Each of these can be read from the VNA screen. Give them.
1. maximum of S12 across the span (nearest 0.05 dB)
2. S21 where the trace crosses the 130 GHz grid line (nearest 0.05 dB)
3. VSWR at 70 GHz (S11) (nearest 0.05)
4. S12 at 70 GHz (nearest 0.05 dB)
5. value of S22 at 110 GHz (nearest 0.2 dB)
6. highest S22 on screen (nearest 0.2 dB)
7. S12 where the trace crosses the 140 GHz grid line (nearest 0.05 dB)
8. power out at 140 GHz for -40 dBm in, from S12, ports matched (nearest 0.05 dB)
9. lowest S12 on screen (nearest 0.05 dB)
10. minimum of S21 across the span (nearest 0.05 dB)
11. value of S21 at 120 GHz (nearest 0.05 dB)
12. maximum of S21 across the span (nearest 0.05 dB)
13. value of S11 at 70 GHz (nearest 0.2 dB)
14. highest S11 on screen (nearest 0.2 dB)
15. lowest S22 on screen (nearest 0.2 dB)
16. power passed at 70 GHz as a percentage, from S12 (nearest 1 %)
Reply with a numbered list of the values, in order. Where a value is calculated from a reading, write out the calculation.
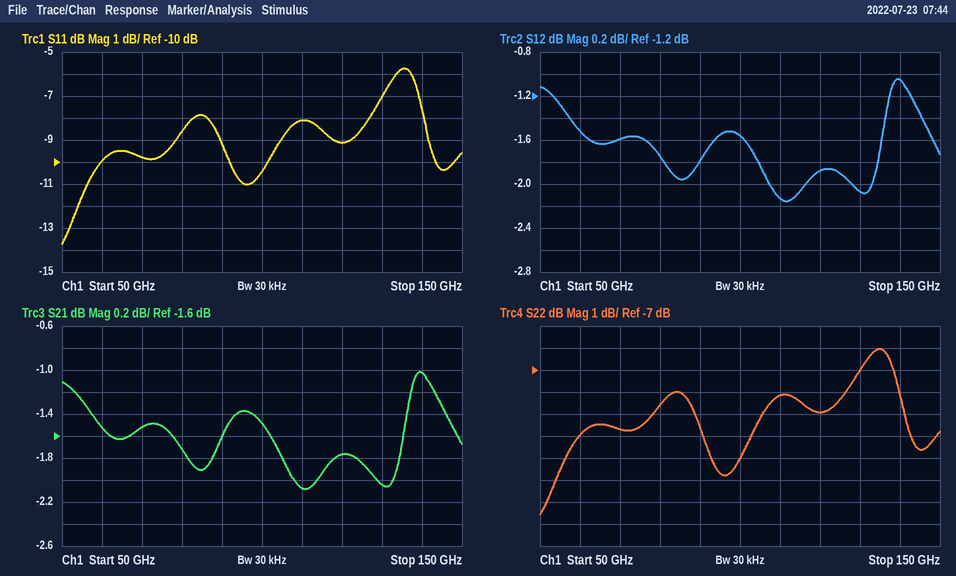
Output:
1. -1.05 dB
2. -2.05 dB
3. |Γ| = 10^(-9.8/20) = 0.3236; VSWR = (1 + 0.3236)/(1 − 0.3236) ≈ 1.96, so 1.95 to the nearest 0.05
4. -1.60 dB
5. -8.2 dB
6. -6.0 dB
7. -1.05 dB
8. -40 dBm + (-1.05 dB) = -41.05 dBm
9. -2.15 dB
10. -2.10 dB
11. -1.75 dB
12. -1.00 dB
13. -9.8 dB
14. -5.8 dB
15. -13.6 dB
16. 10^(-1.6/10) ≈ 69 %
